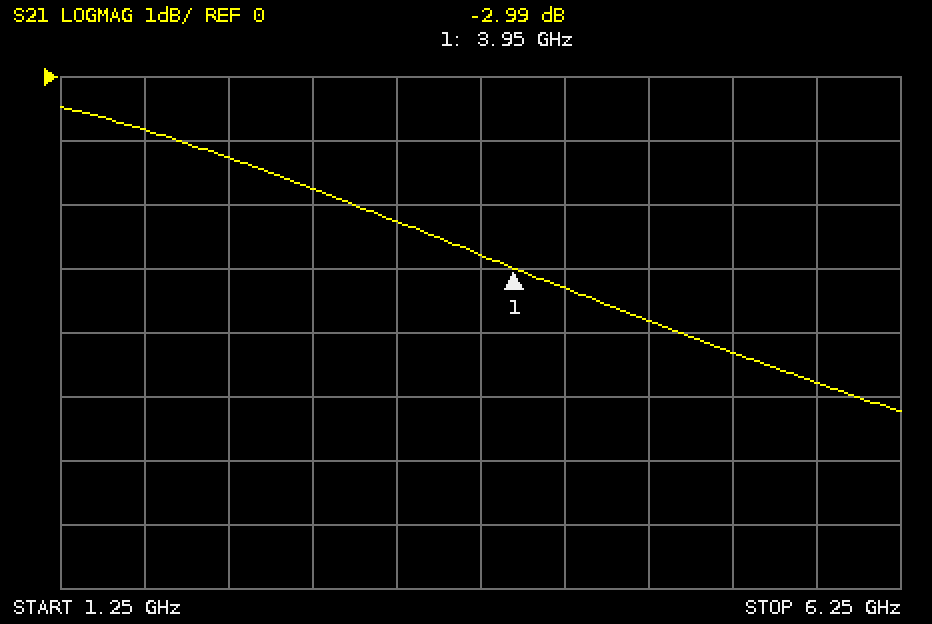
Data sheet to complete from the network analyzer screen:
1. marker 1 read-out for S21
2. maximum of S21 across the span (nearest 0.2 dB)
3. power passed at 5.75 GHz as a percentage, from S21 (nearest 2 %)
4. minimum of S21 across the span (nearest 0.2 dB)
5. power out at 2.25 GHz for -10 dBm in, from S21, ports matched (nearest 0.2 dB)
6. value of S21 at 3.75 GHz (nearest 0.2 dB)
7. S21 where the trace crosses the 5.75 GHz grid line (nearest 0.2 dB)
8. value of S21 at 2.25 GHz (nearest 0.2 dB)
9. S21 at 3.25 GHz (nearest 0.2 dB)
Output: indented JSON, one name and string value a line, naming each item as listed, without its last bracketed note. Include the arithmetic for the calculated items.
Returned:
{
  "marker 1 read-out for S21": "-2.99 dB",
  "maximum of S21 across the span": "-0.4 dB",
  "power passed at 5.75 GHz as a percentage, from S21": "10^(-4.8/10) ≈ 33.1 %, so 34 % to the nearest 2 %",
  "minimum of S21 across the span": "-5.2 dB",
  "power out at 2.25 GHz for -10 dBm in, from S21, ports matched": "-10 dBm + (-1.2 dB) = -11.2 dBm",
  "value of S21 at 3.75 GHz": "-2.8 dB",
  "S21 where the trace crosses the 5.75 GHz grid line": "-4.8 dB",
  "value of S21 at 2.25 GHz": "-1.2 dB",
  "S21 at 3.25 GHz": "-2.2 dB"
}
